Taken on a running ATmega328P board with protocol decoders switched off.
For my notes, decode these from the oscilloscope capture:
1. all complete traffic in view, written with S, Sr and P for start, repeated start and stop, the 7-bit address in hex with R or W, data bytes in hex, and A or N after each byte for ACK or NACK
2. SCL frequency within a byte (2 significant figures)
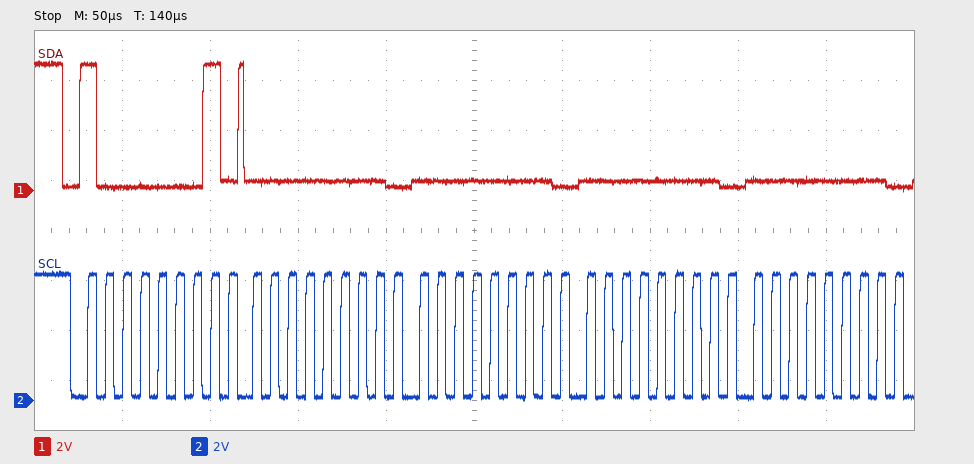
S 40R A 00 A 00 A 00 A 00 A
100 kHz
